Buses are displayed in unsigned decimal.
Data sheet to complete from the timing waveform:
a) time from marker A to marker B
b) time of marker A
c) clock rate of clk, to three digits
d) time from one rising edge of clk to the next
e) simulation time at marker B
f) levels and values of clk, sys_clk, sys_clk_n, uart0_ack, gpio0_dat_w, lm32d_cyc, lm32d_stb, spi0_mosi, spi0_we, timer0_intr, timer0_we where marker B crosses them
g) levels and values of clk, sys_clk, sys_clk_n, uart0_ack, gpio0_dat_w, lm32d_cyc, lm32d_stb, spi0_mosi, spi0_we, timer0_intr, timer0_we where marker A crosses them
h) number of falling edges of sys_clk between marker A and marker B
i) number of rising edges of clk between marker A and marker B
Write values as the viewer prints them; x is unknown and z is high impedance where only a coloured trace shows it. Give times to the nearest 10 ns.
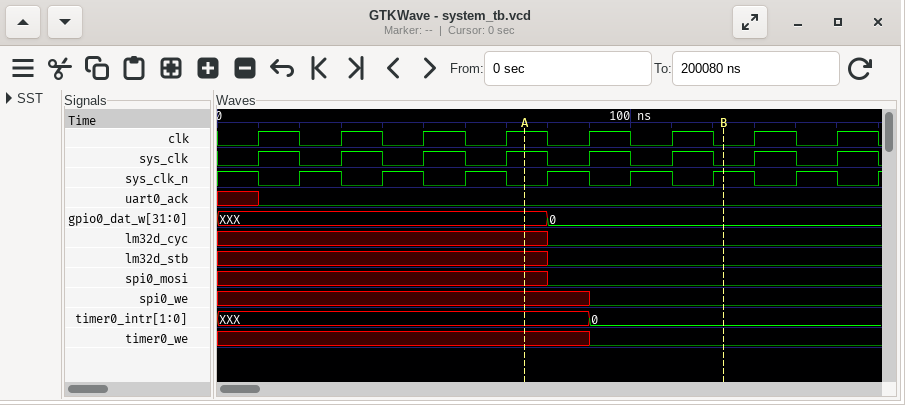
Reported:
50 ns
70 ns
50.0 MHz
20 ns
120 ns
clk=0, sys_clk=0, sys_clk_n=1, uart0_ack=0, gpio0_dat_w=0, lm32d_cyc=0, lm32d_stb=0, spi0_mosi=0, spi0_we=0, timer0_intr=0, timer0_we=0
clk=1, sys_clk=1, sys_clk_n=0, uart0_ack=0, gpio0_dat_w=XXX, lm32d_cyc=x, lm32d_stb=x, spi0_mosi=x, spi0_we=x, timer0_intr=XXX, timer0_we=x
3
2
